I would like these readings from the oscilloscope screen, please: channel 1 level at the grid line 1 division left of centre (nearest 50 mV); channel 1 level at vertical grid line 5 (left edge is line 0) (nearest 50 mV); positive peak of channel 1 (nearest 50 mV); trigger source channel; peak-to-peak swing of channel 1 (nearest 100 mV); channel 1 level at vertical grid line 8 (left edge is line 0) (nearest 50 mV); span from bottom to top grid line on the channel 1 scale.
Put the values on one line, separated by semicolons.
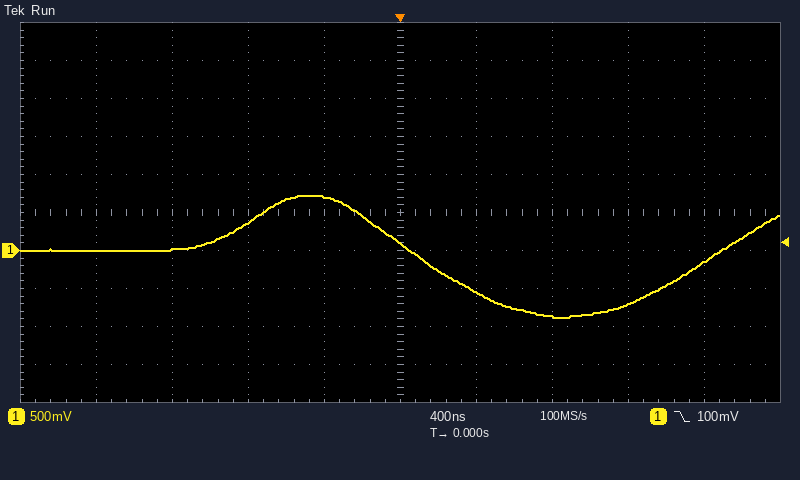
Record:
700 mV; 100 mV; 700 mV; channel 1; 1.60 V; -700 mV; 5 V
